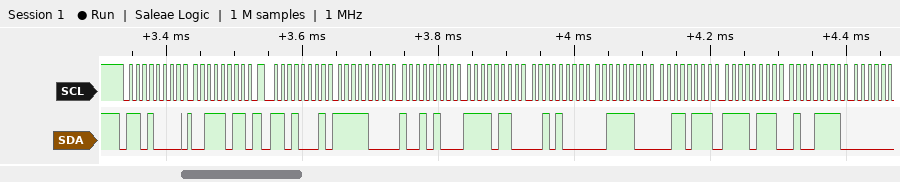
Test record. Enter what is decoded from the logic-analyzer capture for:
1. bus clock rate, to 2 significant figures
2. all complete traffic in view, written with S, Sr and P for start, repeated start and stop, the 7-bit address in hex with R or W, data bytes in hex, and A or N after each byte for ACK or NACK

100 kHz
S 68W A 3B A Sr 68R A F8 A 94 A F6 A 28 A 3C A 37 A F7 A 4F A
